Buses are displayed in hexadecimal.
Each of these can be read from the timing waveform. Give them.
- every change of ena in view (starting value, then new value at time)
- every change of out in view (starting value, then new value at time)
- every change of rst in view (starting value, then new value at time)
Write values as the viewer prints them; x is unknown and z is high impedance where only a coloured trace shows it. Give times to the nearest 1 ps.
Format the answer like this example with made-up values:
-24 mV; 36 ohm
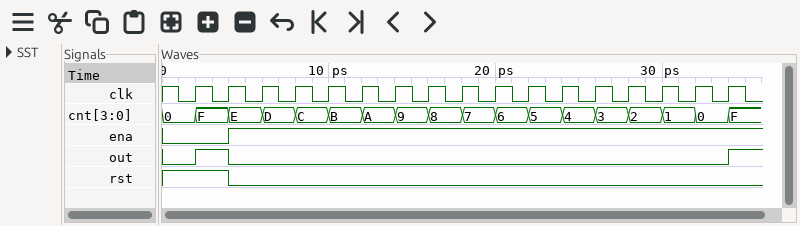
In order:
0, 1 at 4 ps; 0, 1 at 2 ps, 0 at 4 ps, 1 at 34 ps; 1, 0 at 4 ps
